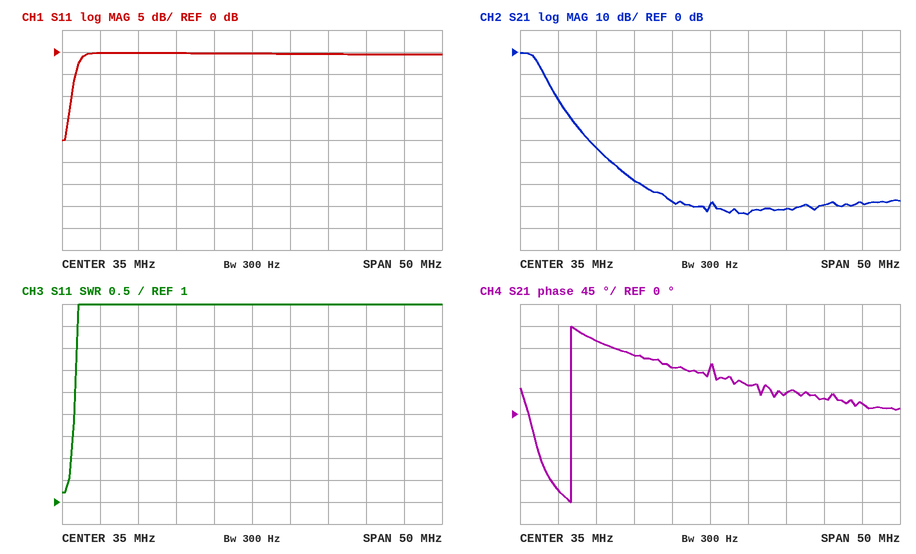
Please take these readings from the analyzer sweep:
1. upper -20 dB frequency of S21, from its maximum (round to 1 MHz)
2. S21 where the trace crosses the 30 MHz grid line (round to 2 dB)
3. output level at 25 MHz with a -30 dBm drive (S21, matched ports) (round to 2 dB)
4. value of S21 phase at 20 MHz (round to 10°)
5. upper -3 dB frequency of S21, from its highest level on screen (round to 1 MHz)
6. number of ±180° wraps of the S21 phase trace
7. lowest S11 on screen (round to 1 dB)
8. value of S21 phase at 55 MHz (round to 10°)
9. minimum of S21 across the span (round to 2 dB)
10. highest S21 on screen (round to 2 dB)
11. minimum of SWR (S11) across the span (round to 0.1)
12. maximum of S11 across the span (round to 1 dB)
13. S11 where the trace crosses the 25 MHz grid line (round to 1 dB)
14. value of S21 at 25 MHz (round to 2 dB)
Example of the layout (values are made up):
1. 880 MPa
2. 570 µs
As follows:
1. 15 MHz
2. -68 dB
3. -88 dBm
4. 150°
5. 12 MHz
6. 1
7. -20 dB
8. 20°
9. -74 dB
10. 0 dB
11. 1.2
12. 0 dB
13. 0 dB
14. -58 dB
